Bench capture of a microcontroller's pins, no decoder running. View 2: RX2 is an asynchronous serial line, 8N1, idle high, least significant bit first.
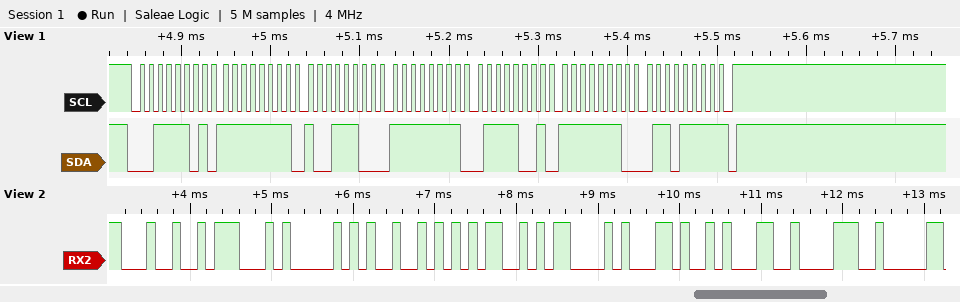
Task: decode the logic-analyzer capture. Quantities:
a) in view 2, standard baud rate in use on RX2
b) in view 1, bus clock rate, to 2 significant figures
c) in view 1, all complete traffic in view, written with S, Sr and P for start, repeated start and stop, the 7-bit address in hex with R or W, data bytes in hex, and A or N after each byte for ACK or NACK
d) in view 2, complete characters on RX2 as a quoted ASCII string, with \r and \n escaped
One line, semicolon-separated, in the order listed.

9600 baud; 100 kHz; S 1ER A FF A 9C A FF A 79 A FE A 6F N P; "$GPRMC,18"
